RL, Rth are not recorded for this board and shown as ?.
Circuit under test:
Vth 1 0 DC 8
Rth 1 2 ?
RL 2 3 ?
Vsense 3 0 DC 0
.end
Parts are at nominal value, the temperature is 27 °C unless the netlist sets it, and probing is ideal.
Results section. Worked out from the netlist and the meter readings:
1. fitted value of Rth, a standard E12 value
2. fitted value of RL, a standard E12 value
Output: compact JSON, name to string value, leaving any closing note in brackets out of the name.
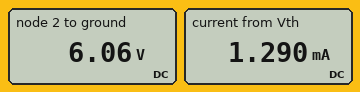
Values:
{"fitted value of Rth, a standard E12 value": "1.5 kΩ", "fitted value of RL, a standard E12 value": "4.7 kΩ"}
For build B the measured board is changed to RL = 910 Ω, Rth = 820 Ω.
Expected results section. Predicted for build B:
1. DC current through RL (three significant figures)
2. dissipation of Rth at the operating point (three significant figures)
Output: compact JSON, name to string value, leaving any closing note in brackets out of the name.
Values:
{"DC current through RL": "4.62 mA", "dissipation of Rth at the operating point": "17.5 mW"}
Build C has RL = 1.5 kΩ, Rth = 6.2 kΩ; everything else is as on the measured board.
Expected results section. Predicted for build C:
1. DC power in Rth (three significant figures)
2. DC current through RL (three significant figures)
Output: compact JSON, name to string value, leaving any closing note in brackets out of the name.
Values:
{"DC power in Rth": "6.69 mW", "DC current through RL": "1.04 mA"}
